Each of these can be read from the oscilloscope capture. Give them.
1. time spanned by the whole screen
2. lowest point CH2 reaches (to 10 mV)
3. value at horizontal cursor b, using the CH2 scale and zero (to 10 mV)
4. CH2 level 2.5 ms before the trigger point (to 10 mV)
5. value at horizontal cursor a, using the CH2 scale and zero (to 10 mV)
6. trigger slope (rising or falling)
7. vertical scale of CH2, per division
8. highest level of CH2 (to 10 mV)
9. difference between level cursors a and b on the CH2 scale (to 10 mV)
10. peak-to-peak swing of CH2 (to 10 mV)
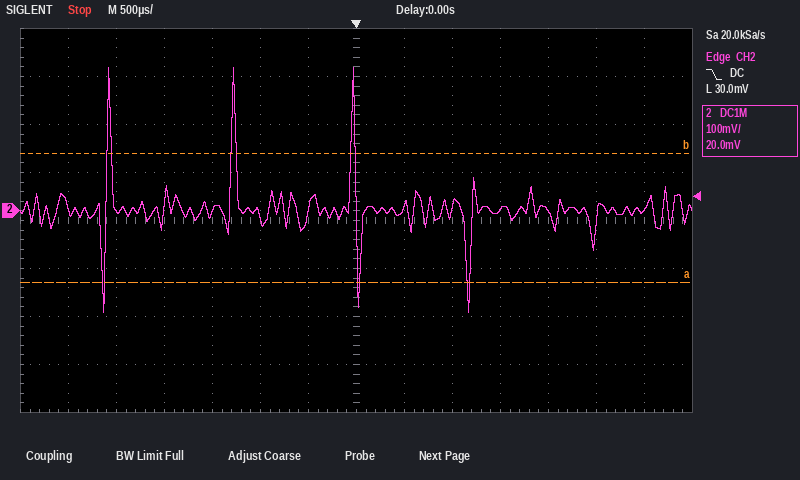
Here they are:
7 ms
-210 mV
120 mV
0 mV
-150 mV
falling
100 mV
300 mV
270 mV
510 mV
